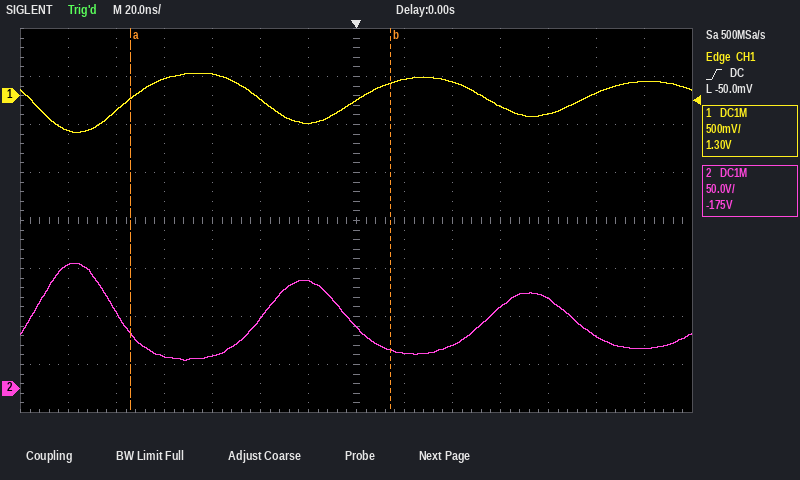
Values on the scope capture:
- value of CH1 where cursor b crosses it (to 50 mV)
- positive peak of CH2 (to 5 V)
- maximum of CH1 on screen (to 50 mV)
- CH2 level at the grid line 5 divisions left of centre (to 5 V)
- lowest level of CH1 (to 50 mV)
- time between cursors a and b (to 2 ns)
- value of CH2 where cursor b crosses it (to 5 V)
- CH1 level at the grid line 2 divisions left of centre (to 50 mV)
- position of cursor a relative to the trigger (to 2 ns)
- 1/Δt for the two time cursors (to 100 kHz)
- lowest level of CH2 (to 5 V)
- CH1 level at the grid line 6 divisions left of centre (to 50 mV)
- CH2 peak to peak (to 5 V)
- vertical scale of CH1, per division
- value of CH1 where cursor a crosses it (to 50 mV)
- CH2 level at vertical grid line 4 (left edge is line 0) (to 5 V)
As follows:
150 mV
130 V
250 mV
80 V
-400 mV
108 ns
40 V
-50 mV
-94 ns
9.3 MHz
30 V
-350 mV
100 V
500 mV
-50 mV
35 V
